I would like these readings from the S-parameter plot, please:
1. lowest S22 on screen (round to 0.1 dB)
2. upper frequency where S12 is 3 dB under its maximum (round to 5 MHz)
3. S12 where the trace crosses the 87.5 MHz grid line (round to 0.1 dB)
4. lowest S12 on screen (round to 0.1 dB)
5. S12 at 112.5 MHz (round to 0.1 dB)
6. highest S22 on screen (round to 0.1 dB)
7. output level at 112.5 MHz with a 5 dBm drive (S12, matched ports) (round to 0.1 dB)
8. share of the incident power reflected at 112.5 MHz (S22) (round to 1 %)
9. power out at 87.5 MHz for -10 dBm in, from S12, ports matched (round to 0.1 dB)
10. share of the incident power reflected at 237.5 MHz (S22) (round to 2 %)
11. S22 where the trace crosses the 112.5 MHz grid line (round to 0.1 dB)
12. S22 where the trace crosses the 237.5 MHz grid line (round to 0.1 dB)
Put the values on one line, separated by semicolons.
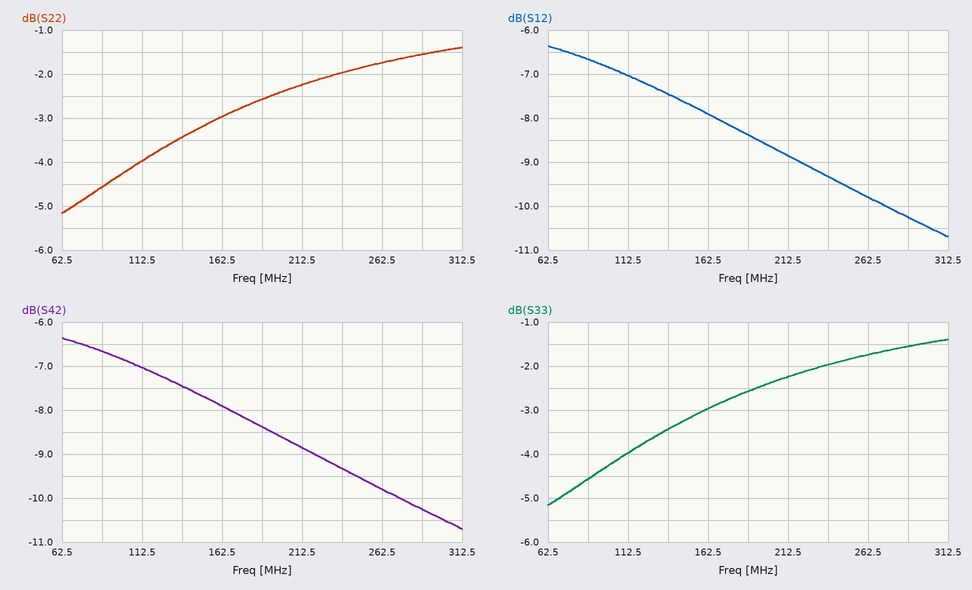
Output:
-5.2 dB; 240 MHz; -6.7 dB; -10.7 dB; -7.0 dB; -1.4 dB; -2.0 dBm; 40 %; -16.7 dBm; 64 %; -4.0 dB; -2.0 dB
